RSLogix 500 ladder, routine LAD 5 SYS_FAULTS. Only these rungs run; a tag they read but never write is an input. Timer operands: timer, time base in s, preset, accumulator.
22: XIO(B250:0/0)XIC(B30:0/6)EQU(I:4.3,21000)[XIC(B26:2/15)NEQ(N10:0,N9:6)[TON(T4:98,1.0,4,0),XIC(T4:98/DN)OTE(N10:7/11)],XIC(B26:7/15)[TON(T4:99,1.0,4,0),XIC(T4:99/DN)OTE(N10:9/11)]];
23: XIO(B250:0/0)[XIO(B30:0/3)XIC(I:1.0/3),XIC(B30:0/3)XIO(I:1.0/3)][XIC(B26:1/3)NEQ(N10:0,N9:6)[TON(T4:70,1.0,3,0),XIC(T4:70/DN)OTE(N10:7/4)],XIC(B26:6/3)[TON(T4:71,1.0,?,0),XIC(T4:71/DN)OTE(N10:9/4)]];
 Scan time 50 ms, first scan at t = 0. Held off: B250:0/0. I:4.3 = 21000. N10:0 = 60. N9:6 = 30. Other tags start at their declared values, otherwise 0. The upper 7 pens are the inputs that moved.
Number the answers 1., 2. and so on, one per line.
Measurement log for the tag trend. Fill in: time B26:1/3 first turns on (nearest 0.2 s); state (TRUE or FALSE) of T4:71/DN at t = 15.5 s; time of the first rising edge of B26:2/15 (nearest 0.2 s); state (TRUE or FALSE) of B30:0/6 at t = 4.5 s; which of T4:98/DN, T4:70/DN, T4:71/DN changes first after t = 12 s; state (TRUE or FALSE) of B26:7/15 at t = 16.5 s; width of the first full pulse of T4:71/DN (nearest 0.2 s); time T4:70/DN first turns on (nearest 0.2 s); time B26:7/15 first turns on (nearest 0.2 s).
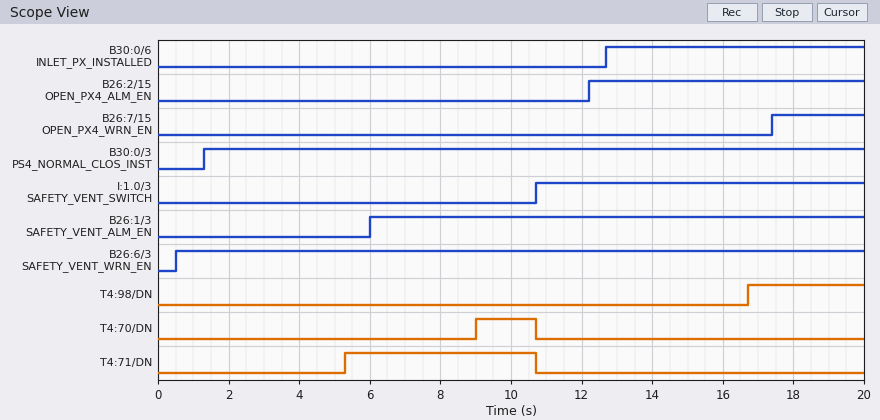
1. 6.0 s
2. FALSE
3. 12.2 s
4. FALSE
5. T4:98/DN
6. FALSE
7. 5.4 s
8. 9.0 s
9. 17.4 s
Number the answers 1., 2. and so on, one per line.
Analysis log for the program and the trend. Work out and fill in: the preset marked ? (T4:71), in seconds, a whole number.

1. 4 s
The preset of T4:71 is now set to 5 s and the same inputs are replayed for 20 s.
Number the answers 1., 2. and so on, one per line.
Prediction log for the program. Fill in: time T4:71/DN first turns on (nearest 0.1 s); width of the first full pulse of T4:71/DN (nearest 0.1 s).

1. 6.3 s
2. 4.4 s
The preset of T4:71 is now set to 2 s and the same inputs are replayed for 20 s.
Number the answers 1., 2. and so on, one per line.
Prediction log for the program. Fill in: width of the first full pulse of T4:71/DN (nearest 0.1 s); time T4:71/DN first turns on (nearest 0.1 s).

1. 7.4 s
2. 3.3 s
